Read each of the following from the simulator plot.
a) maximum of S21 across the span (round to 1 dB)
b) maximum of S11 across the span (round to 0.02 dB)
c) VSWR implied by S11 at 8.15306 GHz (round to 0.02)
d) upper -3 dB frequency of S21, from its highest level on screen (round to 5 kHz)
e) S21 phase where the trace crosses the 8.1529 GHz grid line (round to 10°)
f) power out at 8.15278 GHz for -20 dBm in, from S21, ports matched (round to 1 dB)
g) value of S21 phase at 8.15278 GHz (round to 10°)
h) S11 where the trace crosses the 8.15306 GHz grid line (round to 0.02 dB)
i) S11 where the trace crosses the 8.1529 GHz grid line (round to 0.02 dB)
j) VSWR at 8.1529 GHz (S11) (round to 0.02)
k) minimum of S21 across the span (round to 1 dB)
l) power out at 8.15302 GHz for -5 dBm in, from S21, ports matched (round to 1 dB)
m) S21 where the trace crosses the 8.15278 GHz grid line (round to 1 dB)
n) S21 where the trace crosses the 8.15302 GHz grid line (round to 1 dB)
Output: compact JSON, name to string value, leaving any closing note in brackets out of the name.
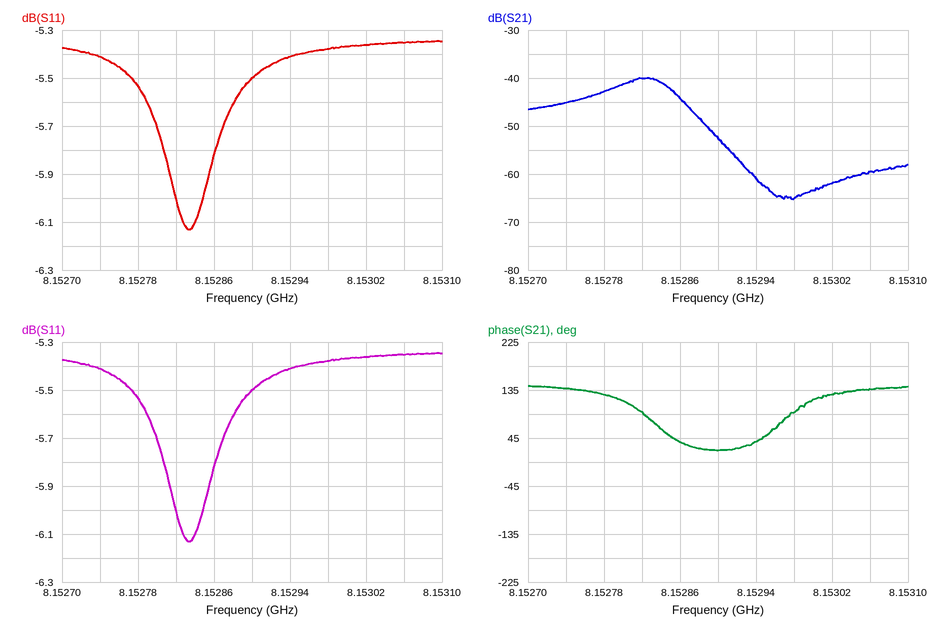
{"maximum of S21 across the span": "-40 dB", "maximum of S11 across the span": "-5.34 dB", "VSWR implied by S11 at 8.15306 GHz": "3.34", "upper -3 dB frequency of S21, from its highest level on screen": "8.152855 GHz", "S21 phase where the trace crosses the 8.1529 GHz grid line": "20°", "power out at 8.15278 GHz for -20 dBm in, from S21, ports matched": "-63 dBm", "value of S21 phase at 8.15278 GHz": "130°", "S11 where the trace crosses the 8.15306 GHz grid line": "-5.36 dB", "S11 where the trace crosses the 8.1529 GHz grid line": "-5.50 dB", "VSWR at 8.1529 GHz (S11)": "3.26", "minimum of S21 across the span": "-65 dB", "power out at 8.15302 GHz for -5 dBm in, from S21, ports matched": "-67 dBm", "S21 where the trace crosses the 8.15278 GHz grid line": "-43 dB", "S21 where the trace crosses the 8.15302 GHz grid line": "-62 dB"}
